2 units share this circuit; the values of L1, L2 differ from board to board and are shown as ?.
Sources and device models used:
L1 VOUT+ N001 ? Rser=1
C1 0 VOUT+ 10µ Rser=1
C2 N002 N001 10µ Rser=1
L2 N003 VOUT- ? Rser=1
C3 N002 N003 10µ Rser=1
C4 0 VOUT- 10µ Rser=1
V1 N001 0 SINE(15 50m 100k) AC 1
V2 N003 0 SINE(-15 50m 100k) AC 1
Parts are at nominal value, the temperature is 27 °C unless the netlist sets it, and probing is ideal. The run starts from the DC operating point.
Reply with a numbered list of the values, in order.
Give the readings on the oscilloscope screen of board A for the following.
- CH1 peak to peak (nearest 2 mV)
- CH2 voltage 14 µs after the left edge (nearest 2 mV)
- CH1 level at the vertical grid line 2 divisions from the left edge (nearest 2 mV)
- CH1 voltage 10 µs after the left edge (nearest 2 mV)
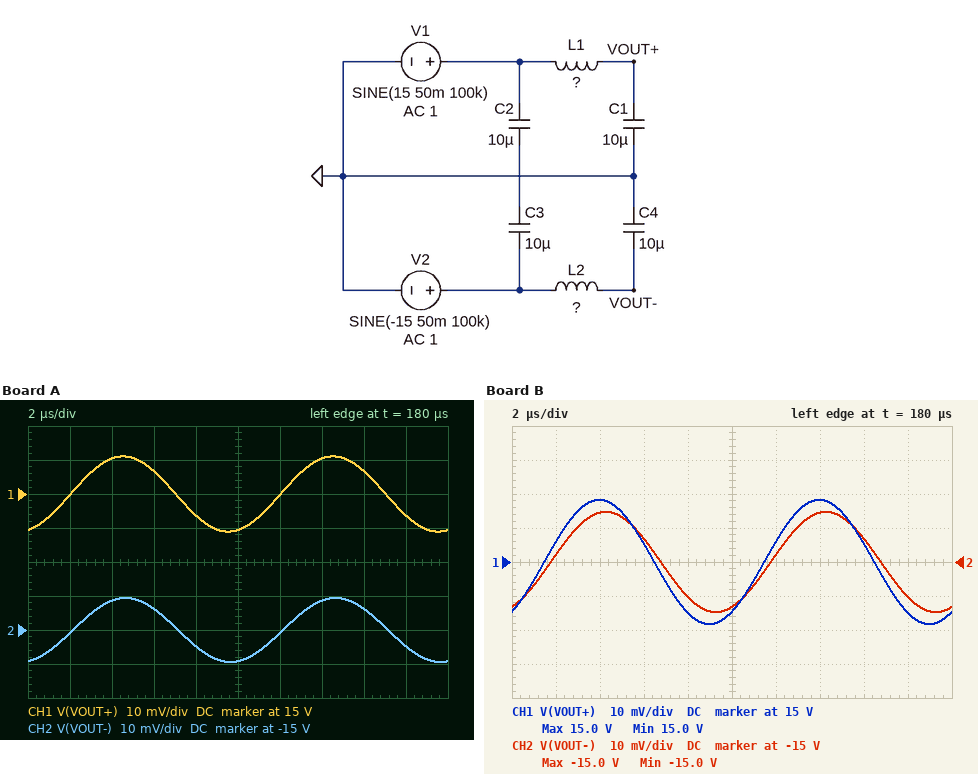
1. 22 mV
2. -14.992 V
3. 15.010 V
4. 14.990 V
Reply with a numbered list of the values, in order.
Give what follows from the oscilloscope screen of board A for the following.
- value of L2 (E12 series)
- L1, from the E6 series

1. 8.2 µH
2. 6.8 µH
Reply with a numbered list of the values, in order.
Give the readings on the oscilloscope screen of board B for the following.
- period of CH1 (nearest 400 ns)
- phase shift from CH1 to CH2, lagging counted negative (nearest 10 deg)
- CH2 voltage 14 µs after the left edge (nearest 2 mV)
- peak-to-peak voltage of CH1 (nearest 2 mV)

1. 10.0 µs
2. -10 deg
3. -14.986 V
4. 36 mV
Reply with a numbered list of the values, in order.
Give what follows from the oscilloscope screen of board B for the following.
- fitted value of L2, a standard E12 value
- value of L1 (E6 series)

1. 4.7 µH
2. 3.3 µH
